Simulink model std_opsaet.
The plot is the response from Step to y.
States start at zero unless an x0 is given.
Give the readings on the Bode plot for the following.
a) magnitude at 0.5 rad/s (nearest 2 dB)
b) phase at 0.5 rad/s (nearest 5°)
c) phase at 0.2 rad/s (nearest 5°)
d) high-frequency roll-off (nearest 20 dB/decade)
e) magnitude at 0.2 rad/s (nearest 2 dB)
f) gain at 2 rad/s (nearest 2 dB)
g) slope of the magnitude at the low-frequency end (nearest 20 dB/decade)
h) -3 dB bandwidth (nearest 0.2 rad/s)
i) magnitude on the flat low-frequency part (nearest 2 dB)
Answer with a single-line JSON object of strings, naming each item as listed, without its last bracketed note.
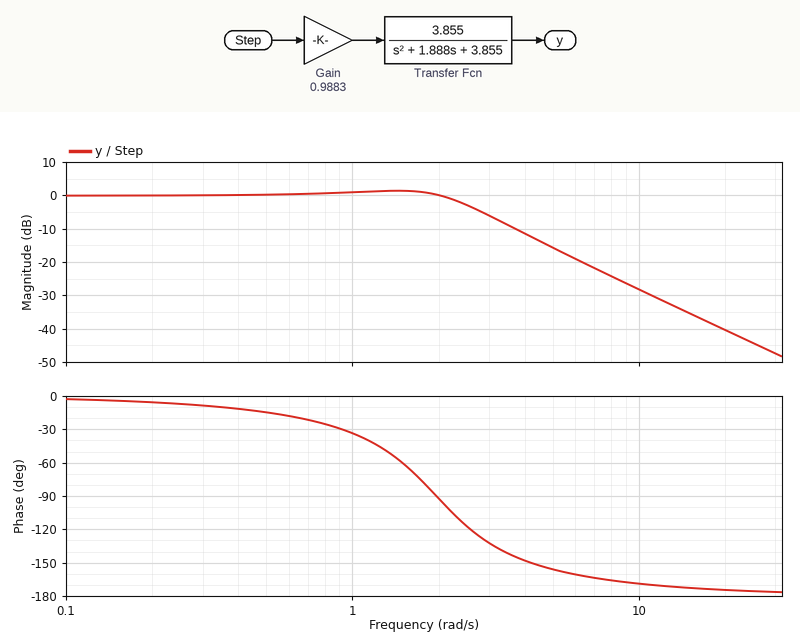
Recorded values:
{"magnitude at 0.5 rad/s": "0 dB", "phase at 0.5 rad/s": "-15°", "phase at 0.2 rad/s": "-5°", "high-frequency roll-off": "-40 dB/decade", "magnitude at 0.2 rad/s": "0 dB", "gain at 2 rad/s": "0 dB", "slope of the magnitude at the low-frequency end": "0 dB/decade", "-3 dB bandwidth": "2.6 rad/s", "magnitude on the flat low-frequency part": "0 dB"}
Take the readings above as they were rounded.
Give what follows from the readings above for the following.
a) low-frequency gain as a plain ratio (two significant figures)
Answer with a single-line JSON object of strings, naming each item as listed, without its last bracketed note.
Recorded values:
{"low-frequency gain as a plain ratio": "1.0"}
